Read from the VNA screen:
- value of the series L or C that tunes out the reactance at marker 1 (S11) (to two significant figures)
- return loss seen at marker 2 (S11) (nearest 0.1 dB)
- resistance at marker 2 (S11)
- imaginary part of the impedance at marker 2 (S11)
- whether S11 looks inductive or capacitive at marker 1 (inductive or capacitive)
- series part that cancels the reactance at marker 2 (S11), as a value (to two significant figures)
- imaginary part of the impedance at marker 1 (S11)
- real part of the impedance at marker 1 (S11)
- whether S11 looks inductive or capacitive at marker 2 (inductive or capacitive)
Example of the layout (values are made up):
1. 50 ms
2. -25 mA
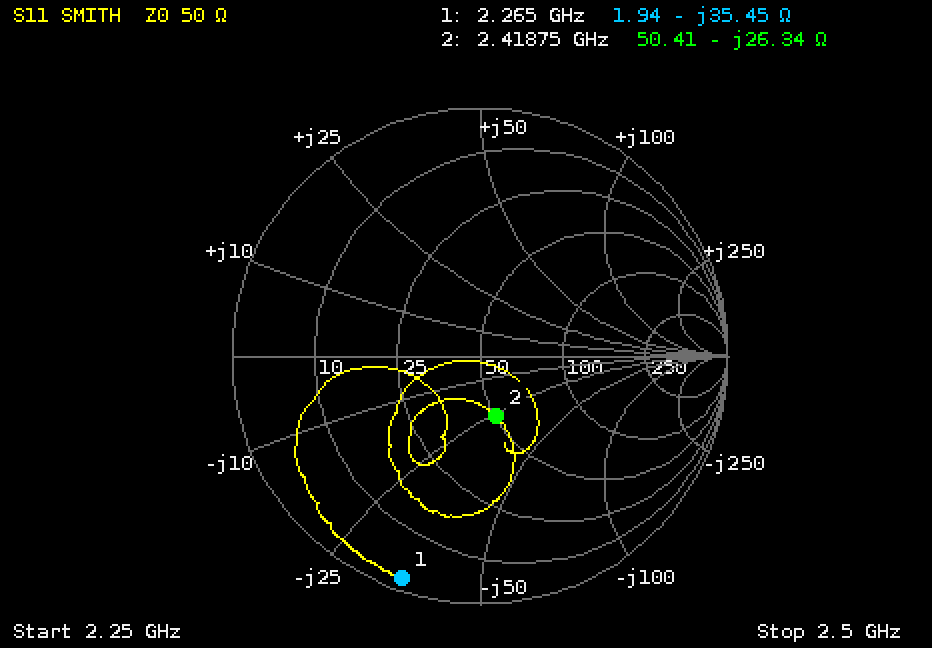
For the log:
1. 2.5 nH
2. 11.9 dB
3. 50.41 Ω
4. -26.34 Ω
5. capacitive
6. 1.7 nH
7. -35.45 Ω
8. 1.94 Ω
9. capacitive
